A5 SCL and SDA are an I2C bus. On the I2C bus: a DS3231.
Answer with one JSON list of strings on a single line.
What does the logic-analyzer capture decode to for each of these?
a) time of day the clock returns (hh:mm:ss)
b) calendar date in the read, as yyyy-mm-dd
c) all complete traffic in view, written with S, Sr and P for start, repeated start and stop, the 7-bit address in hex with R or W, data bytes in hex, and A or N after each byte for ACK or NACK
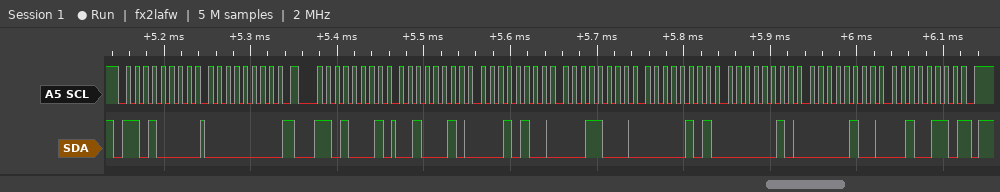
["18:14:22", "2026-04-02", "S 68W A 00 A Sr 68R A 22 A 14 A 18 A 05 A 02 A 04 A 26 N P"]
